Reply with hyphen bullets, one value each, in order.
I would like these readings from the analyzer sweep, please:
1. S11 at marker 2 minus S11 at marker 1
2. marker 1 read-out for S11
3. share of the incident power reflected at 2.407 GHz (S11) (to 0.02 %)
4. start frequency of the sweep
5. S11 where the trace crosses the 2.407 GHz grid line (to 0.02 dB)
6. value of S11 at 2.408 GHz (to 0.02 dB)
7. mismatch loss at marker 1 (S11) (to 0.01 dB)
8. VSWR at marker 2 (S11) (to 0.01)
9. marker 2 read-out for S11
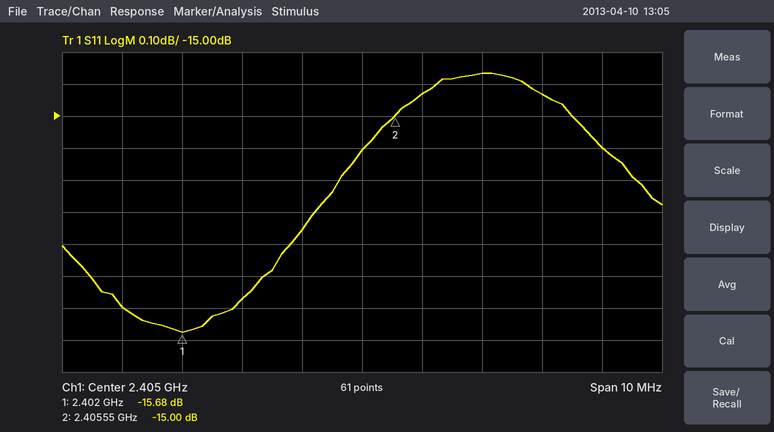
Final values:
- 0.68 dB
- -15.68 dB
- 3.26 %
- 2.4 GHz
- -14.86 dB
- -14.94 dB
- 0.12 dB
- 1.43
- -15.00 dB
